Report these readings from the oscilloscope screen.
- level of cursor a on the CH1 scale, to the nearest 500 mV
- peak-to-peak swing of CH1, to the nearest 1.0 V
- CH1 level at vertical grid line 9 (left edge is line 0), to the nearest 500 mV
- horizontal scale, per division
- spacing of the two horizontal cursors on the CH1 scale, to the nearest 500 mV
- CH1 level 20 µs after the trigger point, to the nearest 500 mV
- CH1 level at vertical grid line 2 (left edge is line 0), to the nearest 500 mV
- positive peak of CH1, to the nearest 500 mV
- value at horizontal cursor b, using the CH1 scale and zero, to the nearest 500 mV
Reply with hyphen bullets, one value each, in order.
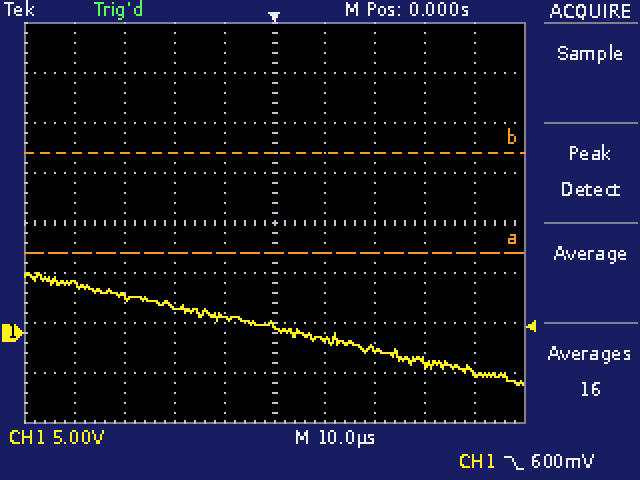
- 8.0 V
- 11.0 V
- -4.0 V
- 10 µs
- 10.0 V
- -1.5 V
- 3.5 V
- 6.0 V
- 18.0 V
